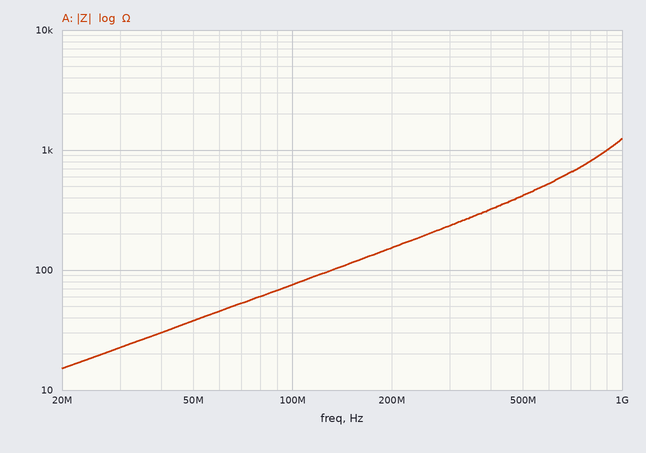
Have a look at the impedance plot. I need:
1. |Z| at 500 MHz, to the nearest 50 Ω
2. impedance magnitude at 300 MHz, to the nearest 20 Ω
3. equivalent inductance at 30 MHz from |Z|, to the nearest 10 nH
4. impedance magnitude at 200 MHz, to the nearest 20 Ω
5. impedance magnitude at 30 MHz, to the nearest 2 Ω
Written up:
400 Ω
240 Ω
120 nH
160 Ω
22 Ω
